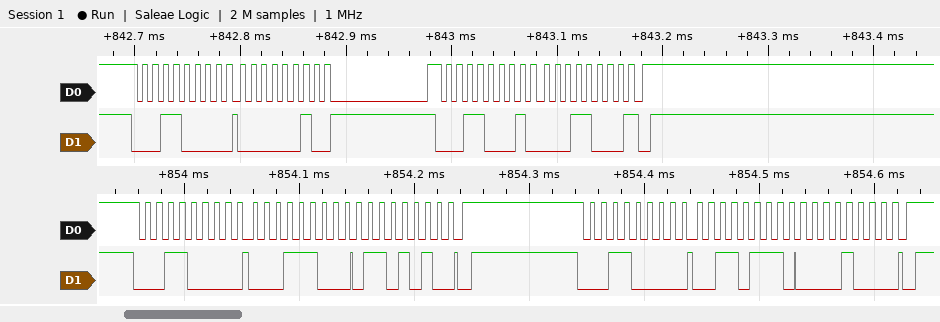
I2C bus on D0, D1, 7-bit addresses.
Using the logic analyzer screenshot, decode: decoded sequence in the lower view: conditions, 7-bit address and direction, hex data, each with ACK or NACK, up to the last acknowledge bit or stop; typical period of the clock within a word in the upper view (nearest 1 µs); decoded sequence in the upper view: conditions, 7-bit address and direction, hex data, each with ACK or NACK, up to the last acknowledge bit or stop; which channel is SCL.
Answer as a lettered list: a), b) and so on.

a) start, address 18 write ACK, 1C ACK, 6A ACK, stop, start, address 18 write ACK, 37 ACK, 08 ACK, stop
b) 10 µs
c) start, address 18 write ACK, 02 ACK, repeated start, address 18 read ACK, 18 NACK, stop
d) D0
